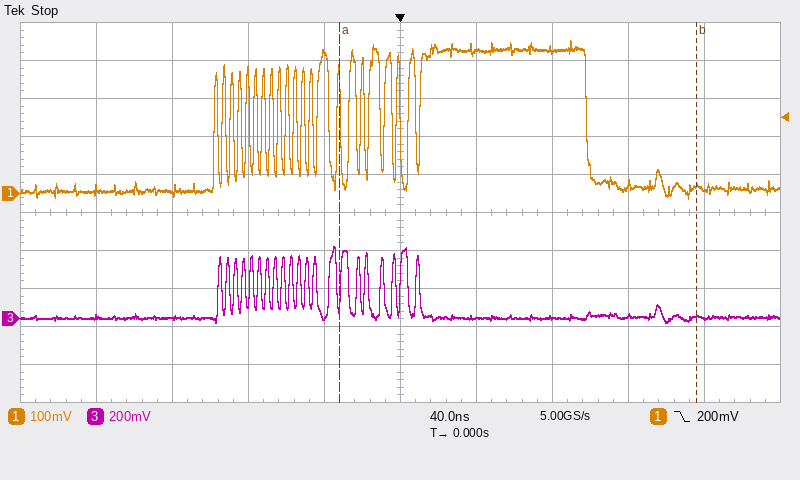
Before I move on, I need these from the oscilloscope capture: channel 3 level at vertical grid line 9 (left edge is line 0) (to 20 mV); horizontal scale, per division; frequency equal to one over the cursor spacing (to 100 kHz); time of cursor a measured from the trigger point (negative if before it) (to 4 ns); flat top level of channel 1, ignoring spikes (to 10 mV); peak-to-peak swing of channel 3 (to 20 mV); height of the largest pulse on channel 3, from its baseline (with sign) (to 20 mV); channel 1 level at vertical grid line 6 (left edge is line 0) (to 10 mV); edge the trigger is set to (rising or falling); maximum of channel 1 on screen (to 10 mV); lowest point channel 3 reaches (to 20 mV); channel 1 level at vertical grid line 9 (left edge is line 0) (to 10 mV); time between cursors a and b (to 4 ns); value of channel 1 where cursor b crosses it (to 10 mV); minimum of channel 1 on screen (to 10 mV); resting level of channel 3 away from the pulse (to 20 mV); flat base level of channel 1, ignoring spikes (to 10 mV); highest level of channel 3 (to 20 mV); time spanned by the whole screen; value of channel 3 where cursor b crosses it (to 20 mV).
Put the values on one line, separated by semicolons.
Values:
0 mV; 40 ns; 5.3 MHz; -32 ns; 380 mV; 400 mV; +380 mV; 370 mV; falling; 400 mV; -20 mV; 10 mV; 188 ns; 20 mV; -10 mV; 0 mV; 10 mV; 380 mV; 400 ns; 20 mV
